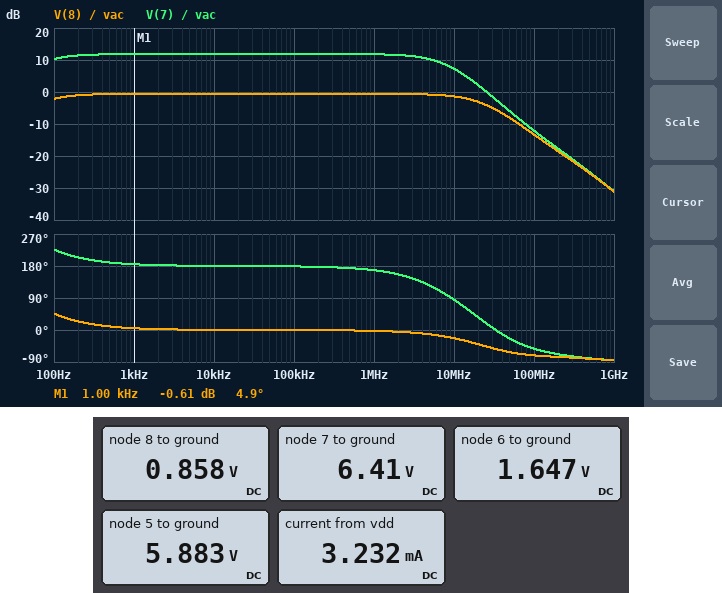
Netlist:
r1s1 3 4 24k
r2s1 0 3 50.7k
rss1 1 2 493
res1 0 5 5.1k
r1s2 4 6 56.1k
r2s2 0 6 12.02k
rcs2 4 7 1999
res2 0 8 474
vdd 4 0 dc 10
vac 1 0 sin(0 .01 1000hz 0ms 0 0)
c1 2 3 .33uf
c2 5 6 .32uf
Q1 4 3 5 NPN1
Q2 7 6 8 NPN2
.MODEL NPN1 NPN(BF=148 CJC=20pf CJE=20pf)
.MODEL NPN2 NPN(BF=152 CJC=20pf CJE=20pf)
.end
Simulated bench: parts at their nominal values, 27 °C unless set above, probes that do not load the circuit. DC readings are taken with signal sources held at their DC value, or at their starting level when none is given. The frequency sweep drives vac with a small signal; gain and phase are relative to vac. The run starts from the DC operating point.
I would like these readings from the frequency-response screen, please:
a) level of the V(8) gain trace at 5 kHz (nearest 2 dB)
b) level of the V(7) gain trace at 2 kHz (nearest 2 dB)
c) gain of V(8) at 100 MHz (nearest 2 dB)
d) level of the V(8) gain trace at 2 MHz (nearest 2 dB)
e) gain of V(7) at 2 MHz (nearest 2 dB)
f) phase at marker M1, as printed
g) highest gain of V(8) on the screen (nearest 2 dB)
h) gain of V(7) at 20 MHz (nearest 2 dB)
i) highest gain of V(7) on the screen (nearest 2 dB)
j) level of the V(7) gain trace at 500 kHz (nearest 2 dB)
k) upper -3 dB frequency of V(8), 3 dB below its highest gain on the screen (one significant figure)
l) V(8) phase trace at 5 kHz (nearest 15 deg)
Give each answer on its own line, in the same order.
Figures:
0 dB
12 dB
-14 dB
0 dB
12 dB
4.9 deg
0 dB
2 dB
12 dB
12 dB
20 MHz
0 deg
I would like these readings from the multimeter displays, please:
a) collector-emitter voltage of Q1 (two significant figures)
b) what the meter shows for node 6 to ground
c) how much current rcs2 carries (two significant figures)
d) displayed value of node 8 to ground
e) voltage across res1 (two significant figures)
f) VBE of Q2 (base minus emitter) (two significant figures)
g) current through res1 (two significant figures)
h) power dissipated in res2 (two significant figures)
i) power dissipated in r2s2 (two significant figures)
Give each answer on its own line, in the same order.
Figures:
4.1 V
1.647 V
1.8 mA
0.858 V
5.9 V
790 mV
1.2 mA
1.6 mW
230 µW
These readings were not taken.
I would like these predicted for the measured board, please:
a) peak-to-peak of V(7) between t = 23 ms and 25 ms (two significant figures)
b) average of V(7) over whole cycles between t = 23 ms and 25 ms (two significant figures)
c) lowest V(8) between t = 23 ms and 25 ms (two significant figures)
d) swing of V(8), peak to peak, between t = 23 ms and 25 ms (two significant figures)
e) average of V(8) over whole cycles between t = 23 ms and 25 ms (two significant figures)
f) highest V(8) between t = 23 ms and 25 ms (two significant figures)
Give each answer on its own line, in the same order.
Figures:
78 mV
6.4 V
850 mV
19 mV
860 mV
870 mV
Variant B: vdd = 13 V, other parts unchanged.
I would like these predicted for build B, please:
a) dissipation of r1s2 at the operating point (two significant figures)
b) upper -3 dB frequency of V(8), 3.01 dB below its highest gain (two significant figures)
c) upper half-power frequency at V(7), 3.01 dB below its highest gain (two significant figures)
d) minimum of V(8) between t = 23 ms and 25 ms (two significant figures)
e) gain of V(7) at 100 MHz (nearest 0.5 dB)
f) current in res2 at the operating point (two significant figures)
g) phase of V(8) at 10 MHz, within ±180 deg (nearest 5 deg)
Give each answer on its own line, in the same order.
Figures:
2.1 mW
26 MHz
7.7 MHz
1.3 V
-11.5 dB
2.8 mA
-20 deg
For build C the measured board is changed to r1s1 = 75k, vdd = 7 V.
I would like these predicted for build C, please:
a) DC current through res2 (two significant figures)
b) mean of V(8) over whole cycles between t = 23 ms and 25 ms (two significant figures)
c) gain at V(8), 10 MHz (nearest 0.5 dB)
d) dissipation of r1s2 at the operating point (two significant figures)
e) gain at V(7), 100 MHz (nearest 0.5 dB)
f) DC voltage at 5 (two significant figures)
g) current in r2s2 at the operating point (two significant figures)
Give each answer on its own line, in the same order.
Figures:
860 µA
410 mV
-2.5 dB
600 µW
-12.5 dB
2.0 V
98 µA
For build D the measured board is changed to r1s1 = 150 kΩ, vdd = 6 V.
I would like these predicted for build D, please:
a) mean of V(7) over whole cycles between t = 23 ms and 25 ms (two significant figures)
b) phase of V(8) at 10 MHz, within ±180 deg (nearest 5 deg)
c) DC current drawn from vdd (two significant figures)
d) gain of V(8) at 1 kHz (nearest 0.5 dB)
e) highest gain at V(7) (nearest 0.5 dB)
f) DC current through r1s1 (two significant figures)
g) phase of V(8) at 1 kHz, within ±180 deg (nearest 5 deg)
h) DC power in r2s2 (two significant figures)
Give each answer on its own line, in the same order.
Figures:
4.9 V
-35 deg
820 µA
-1.5 dB
11.0 dB
30 µA
5 deg
87 µW
